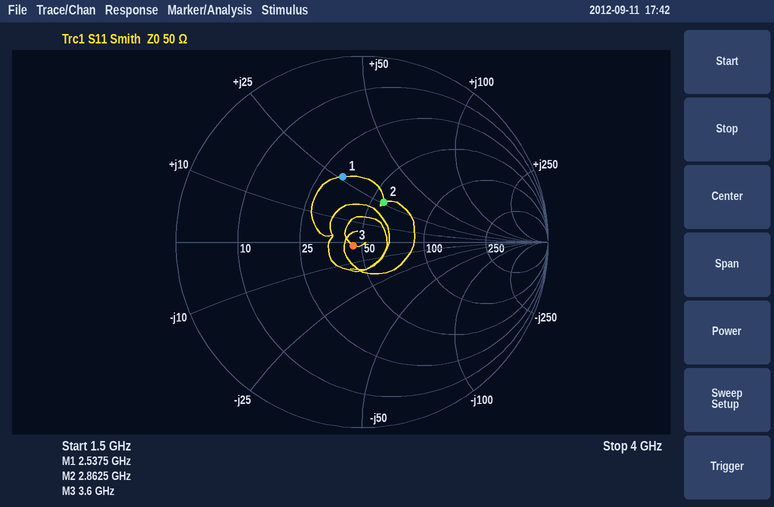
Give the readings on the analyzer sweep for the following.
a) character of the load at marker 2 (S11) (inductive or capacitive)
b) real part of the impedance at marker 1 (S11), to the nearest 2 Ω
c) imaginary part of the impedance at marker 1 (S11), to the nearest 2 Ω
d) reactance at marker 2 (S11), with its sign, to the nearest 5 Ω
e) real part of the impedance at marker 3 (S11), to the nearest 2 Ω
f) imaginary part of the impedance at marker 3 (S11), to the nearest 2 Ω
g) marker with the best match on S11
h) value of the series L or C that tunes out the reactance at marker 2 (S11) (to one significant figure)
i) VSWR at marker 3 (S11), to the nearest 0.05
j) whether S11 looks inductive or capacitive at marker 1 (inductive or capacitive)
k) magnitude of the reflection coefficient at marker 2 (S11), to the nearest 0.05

inductive
32 Ω
+26 Ω
+25 Ω
46 Ω
-2 Ω
marker 3
2 pF
1.10
inductive
0.25
